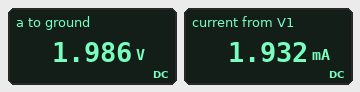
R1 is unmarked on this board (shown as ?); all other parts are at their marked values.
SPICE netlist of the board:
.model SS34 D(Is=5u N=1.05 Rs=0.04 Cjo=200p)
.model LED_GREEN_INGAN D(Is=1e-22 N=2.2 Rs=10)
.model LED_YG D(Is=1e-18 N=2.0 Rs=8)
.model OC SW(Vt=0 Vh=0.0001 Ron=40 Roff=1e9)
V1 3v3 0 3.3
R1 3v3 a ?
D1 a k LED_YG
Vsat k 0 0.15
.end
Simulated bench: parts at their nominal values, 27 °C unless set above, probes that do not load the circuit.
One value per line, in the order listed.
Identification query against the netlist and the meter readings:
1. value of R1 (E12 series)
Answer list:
680 Ω
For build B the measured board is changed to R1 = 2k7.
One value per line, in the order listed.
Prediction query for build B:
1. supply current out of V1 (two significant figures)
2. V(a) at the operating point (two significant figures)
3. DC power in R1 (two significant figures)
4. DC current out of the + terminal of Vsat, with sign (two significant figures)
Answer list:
520 µA
1.9 V
720 µW
-520 µA
